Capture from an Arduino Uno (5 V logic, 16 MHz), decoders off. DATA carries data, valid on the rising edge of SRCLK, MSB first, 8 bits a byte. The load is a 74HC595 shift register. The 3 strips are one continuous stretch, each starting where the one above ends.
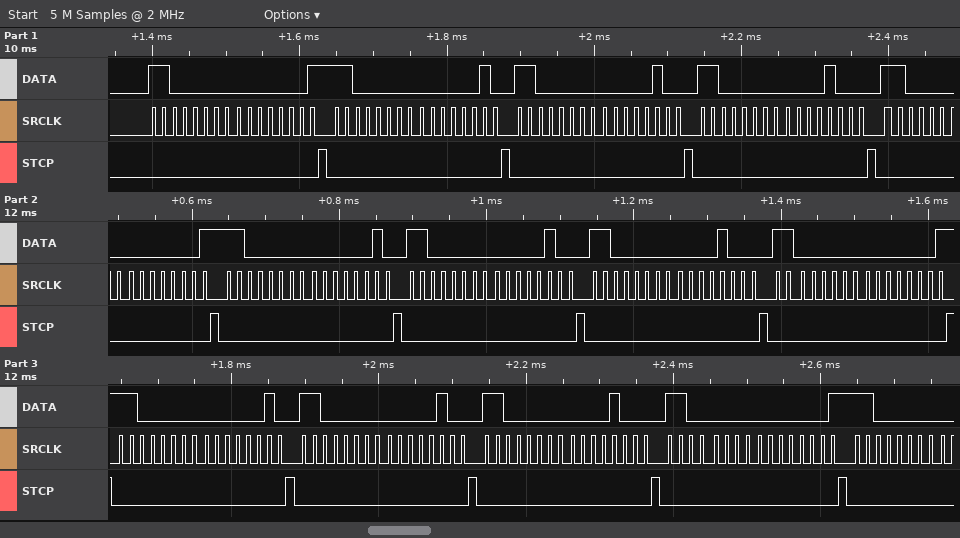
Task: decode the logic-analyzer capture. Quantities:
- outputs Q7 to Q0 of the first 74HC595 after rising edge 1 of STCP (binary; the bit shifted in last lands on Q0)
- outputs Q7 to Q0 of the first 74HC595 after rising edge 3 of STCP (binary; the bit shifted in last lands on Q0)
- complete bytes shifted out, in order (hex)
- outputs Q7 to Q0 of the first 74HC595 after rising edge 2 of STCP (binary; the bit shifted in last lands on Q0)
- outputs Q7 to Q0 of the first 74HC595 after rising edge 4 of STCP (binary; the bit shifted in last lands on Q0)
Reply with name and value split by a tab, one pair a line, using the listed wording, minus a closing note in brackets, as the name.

outputs Q7 to Q0 of the first 74HC595 after rising edge 1 of STCP	00000001
outputs Q7 to Q0 of the first 74HC595 after rising edge 3 of STCP	00000100
complete bytes shifted out, in order	C0 01 C0 02 C0 04 C0 08 C0 01 C0 02 C0 04 C0 08 C0 01 C0 02 C0 04 C0 08 C0 01 C0
outputs Q7 to Q0 of the first 74HC595 after rising edge 2 of STCP	00000010
outputs Q7 to Q0 of the first 74HC595 after rising edge 4 of STCP	00001000
